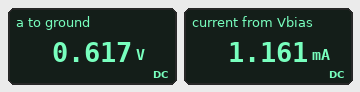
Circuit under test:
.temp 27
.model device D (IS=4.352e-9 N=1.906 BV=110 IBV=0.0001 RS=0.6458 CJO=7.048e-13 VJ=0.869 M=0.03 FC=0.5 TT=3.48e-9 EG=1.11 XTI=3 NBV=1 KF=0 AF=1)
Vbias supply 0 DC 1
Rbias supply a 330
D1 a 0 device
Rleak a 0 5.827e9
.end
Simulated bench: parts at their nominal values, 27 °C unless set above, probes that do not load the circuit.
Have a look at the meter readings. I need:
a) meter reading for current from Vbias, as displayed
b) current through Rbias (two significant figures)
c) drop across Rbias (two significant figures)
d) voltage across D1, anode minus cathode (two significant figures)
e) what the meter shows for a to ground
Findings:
1.161 mA
1.2 mA
380 mV
620 mV
0.617 V
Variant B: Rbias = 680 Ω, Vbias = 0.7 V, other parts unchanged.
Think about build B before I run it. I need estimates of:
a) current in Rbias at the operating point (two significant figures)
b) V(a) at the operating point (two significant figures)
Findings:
240 µA
540 mV
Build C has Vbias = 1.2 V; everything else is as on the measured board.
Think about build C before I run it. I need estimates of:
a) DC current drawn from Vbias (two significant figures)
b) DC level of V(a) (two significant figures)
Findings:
1.7 mA
640 mV
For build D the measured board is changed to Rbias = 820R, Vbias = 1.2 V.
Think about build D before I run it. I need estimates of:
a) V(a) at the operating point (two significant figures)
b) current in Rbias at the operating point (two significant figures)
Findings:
590 mV
740 µA
